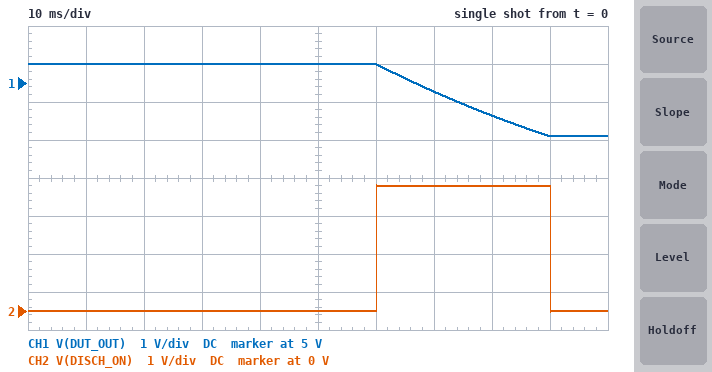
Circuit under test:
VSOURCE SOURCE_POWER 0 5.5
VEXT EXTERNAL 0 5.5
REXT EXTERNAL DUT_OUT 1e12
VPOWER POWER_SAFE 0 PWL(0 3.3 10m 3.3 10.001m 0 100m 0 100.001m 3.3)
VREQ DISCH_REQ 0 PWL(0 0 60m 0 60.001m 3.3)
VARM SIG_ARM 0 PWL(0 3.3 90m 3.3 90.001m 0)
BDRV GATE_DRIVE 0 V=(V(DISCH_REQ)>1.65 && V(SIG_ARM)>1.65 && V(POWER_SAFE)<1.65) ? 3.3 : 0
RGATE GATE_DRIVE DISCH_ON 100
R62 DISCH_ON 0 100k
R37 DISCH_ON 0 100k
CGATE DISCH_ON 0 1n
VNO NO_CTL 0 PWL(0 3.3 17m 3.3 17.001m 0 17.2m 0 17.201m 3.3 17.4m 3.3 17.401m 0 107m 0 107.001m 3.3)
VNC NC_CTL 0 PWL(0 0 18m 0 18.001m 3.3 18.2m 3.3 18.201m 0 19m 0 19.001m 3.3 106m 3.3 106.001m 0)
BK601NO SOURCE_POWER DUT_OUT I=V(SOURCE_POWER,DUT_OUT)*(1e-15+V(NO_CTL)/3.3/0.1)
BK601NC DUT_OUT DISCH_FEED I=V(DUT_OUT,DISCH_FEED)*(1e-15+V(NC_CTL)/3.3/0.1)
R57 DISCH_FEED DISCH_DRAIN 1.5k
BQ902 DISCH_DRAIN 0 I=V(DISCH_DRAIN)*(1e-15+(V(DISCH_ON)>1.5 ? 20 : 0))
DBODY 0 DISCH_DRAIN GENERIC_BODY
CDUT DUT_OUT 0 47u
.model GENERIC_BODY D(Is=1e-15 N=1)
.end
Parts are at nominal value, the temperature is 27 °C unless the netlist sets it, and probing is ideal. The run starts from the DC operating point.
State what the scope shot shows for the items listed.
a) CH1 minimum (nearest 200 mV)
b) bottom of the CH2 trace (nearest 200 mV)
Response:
3.6 V
0 V
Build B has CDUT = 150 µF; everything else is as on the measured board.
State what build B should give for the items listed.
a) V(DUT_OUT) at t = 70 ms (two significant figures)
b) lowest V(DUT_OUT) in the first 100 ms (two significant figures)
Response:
5.3 V
4.8 V
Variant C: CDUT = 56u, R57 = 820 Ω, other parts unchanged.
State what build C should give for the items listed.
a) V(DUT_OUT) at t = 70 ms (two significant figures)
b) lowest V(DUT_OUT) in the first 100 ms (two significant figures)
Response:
4.4 V
2.9 V
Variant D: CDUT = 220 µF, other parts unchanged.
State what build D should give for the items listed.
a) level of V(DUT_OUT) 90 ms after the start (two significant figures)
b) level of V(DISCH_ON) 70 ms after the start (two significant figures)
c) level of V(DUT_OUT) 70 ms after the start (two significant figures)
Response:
5.0 V
3.3 V
5.3 V
